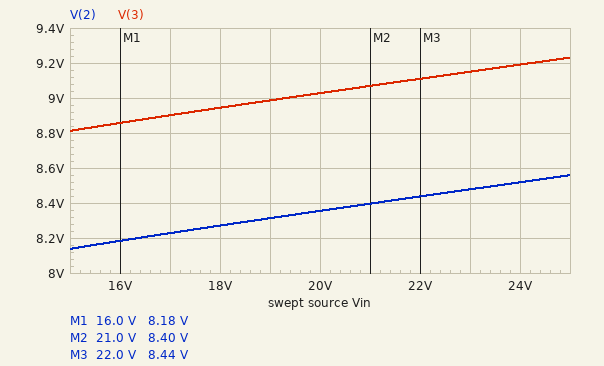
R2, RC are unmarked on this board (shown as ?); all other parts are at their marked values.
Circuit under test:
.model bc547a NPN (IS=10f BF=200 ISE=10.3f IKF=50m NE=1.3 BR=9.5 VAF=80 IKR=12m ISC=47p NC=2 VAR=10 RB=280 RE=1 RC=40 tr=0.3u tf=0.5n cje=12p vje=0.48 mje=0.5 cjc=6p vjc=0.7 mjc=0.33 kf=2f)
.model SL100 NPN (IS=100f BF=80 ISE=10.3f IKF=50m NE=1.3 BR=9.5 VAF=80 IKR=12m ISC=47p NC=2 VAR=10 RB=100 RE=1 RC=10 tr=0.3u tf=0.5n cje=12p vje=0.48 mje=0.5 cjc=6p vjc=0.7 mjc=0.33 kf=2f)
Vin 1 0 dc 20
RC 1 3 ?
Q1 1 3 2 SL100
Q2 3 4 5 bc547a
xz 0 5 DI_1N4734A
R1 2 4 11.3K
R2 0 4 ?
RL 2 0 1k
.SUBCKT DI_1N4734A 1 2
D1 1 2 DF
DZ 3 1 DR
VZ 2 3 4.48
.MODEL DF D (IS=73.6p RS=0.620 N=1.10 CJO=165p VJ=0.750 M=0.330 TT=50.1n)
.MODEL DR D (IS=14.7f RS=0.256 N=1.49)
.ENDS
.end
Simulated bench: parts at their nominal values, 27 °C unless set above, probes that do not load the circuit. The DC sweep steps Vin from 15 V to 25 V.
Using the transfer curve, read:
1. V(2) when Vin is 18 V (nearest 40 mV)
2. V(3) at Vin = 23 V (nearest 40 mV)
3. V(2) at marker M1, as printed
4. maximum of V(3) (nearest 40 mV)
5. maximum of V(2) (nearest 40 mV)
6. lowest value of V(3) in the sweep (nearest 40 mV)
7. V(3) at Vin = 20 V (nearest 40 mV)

8.28 V
9.16 V
8.18 V
9.24 V
8.56 V
8.80 V
9.04 V
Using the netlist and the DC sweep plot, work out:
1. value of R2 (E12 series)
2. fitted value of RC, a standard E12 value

39 kΩ
2.7 kΩ
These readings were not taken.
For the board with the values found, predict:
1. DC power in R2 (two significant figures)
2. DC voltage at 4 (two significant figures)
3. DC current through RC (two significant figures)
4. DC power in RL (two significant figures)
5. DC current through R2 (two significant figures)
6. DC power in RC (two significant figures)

990 µW
6.2 V
4.1 mA
70 mW
160 µA
45 mW
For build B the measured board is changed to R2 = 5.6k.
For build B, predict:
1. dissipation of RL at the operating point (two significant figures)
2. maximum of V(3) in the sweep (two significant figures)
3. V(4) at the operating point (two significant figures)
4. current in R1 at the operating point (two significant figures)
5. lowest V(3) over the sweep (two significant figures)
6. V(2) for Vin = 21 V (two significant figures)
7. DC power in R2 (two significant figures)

320 mW
19 V
6.0 V
1.1 mA
14 V
18 V
6.3 mW
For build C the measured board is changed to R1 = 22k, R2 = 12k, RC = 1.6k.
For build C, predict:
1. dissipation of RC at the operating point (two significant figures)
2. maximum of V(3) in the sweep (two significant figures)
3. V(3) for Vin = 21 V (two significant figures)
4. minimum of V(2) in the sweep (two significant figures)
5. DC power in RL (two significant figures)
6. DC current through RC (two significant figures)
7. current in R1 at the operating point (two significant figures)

2.2 mW
19 V
18 V
14 V
300 mW
1.2 mA
510 µA
